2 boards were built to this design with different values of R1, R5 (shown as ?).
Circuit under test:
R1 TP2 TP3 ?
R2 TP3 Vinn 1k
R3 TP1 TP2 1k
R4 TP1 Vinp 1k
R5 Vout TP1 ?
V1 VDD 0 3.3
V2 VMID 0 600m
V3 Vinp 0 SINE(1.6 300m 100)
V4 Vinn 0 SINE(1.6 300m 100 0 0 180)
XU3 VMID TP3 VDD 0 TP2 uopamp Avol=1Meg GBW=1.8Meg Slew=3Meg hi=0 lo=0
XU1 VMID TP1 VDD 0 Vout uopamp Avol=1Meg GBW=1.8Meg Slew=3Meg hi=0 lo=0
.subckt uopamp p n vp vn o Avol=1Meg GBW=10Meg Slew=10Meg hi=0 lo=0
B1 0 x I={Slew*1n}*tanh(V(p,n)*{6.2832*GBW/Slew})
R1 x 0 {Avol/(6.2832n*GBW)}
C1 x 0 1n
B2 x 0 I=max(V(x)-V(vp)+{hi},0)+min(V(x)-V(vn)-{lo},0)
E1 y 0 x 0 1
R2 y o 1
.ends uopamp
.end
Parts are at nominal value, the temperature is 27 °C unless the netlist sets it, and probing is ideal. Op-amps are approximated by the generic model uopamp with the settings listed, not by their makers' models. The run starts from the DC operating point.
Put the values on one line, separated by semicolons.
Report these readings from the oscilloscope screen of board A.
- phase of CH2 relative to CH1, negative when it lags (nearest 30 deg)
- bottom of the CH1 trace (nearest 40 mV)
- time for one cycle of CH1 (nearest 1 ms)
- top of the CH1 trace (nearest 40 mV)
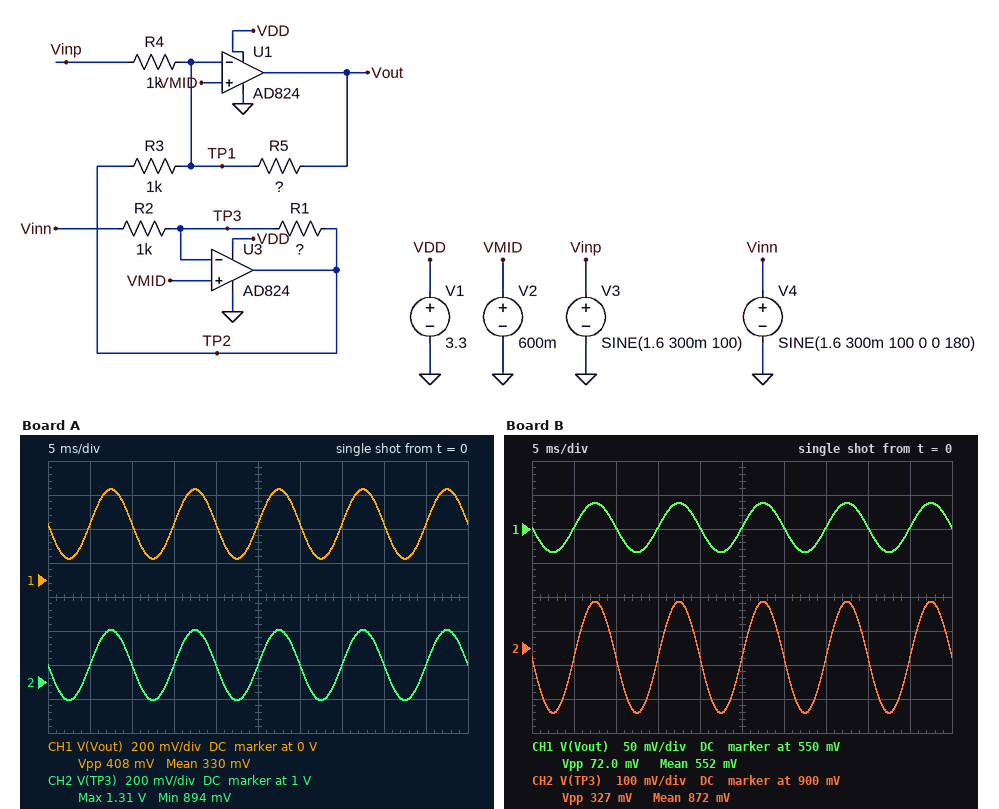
0 deg; 120 mV; 10 ms; 520 mV
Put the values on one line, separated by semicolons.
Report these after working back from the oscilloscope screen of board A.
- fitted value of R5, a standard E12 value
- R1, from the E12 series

680 Ω; 2.2 kΩ
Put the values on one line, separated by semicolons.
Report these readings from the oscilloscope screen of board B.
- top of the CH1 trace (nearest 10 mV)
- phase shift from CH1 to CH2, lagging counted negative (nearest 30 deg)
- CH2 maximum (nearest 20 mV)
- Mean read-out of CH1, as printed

590 mV; 0 deg; 1.04 V; 552 mV
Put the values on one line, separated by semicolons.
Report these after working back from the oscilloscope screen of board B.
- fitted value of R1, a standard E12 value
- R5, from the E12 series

1.2 kΩ; 120 Ω
